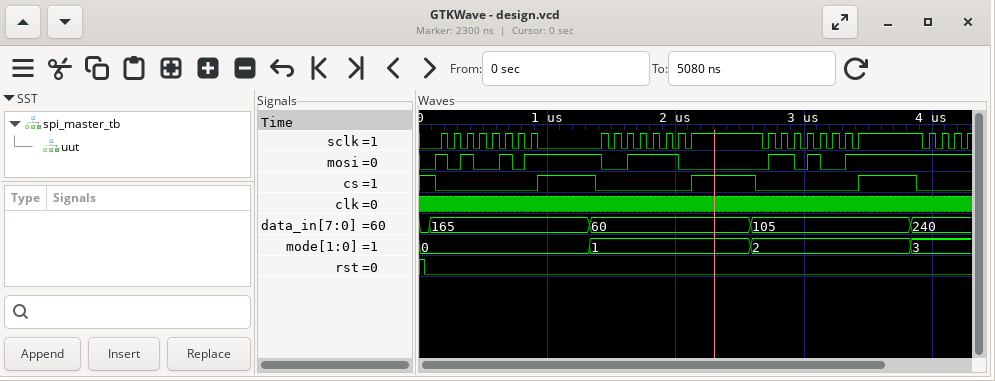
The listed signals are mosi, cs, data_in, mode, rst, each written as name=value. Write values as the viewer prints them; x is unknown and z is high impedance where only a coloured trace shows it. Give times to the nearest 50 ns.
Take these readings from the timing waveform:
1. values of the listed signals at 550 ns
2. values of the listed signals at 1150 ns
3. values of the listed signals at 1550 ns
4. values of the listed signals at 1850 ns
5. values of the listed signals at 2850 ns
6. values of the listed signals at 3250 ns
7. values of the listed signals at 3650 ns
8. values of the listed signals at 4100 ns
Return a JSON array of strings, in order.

["mosi=0, cs=0, data_in=165, mode=0, rst=0", "mosi=1, cs=1, data_in=165, mode=0, rst=0", "mosi=0, cs=0, data_in=60, mode=1, rst=0", "mosi=1, cs=0, data_in=60, mode=1, rst=0", "mosi=1, cs=0, data_in=105, mode=2, rst=0", "mosi=0, cs=0, data_in=105, mode=2, rst=0", "mosi=1, cs=1, data_in=105, mode=2, rst=0", "mosi=1, cs=0, data_in=240, mode=3, rst=0"]
